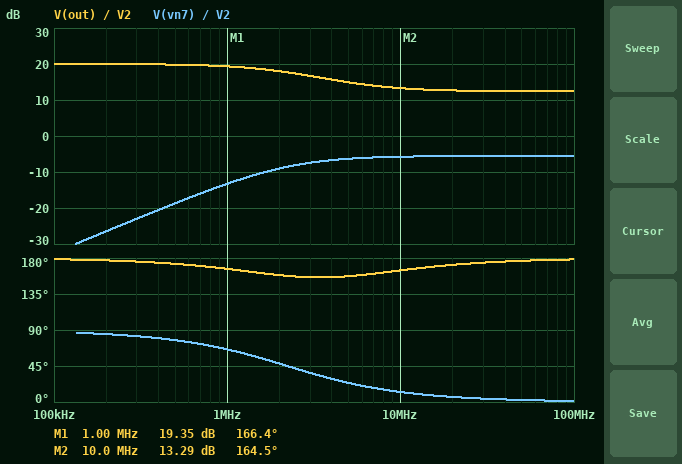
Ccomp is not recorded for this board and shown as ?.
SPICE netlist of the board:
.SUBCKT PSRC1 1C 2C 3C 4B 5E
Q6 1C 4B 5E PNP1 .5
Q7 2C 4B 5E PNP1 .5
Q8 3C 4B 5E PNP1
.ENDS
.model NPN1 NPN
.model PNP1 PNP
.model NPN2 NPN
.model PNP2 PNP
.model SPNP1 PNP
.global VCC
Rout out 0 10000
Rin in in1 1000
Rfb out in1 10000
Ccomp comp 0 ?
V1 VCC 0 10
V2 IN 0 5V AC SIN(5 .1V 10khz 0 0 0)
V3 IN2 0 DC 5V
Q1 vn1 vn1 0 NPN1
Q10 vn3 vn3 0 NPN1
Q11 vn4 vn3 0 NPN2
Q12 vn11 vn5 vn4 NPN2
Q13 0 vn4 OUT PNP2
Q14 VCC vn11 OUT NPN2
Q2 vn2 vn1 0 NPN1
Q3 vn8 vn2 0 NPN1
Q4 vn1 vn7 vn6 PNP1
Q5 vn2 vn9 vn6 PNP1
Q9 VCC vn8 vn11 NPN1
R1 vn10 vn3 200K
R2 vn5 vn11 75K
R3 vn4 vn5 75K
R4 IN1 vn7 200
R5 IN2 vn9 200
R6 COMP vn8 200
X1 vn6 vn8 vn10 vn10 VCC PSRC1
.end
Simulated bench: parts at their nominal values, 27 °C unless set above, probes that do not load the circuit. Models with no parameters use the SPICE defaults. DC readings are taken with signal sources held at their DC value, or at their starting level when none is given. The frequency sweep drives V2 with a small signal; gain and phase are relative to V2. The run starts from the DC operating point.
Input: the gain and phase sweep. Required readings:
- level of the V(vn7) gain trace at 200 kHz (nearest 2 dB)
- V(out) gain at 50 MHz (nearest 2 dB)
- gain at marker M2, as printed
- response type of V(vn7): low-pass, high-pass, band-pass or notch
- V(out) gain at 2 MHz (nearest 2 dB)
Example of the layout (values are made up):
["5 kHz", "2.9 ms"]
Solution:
["-26 dB", "12 dB", "13.29 dB", "high-pass", "18 dB"]
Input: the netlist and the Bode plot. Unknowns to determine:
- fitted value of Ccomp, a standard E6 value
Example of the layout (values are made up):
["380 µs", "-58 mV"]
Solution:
["150 pF"]
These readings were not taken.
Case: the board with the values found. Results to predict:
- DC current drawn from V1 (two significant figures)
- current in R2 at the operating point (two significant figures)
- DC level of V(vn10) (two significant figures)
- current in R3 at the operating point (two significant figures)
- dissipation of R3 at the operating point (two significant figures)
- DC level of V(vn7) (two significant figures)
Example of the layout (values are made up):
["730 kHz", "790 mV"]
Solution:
["630 µA", "9.5 µA", "9.3 V", "9.1 µA", "6.3 µW", "5.0 V"]
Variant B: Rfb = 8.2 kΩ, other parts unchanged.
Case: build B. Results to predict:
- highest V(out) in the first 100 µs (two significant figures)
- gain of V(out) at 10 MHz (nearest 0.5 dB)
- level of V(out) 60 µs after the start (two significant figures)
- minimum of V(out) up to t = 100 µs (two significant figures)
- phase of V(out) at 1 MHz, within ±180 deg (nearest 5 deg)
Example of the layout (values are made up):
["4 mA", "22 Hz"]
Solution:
["5.8 V", "12.5 dB", "5.5 V", "4.2 V", "170 deg"]
